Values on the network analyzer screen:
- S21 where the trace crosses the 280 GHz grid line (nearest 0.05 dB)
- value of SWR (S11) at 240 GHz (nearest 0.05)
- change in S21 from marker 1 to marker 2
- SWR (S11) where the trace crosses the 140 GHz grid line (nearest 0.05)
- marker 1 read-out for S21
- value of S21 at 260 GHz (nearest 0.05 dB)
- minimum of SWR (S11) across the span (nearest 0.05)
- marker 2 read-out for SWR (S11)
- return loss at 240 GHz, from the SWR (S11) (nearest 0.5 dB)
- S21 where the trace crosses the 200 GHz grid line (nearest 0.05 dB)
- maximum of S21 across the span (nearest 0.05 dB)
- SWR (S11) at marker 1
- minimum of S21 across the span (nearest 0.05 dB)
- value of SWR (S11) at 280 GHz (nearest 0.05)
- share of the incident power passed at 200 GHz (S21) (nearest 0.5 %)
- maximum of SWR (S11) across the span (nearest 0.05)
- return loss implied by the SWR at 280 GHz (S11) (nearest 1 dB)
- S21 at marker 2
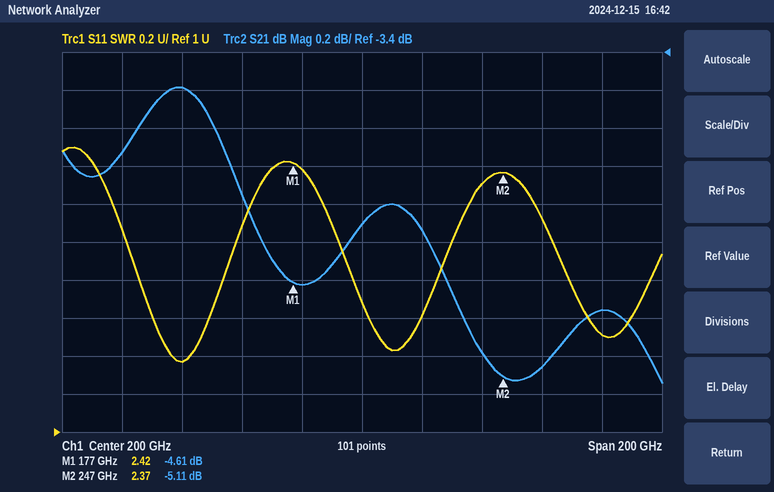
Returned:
-4.75 dB
2.30
-0.50 dB
1.35
-4.61 dB
-5.05 dB
1.35
2.37
8.0 dB
-4.30 dB
-3.60 dB
2.42
-5.15 dB
1.50
37.0 %
2.50
14 dB
-5.11 dB
